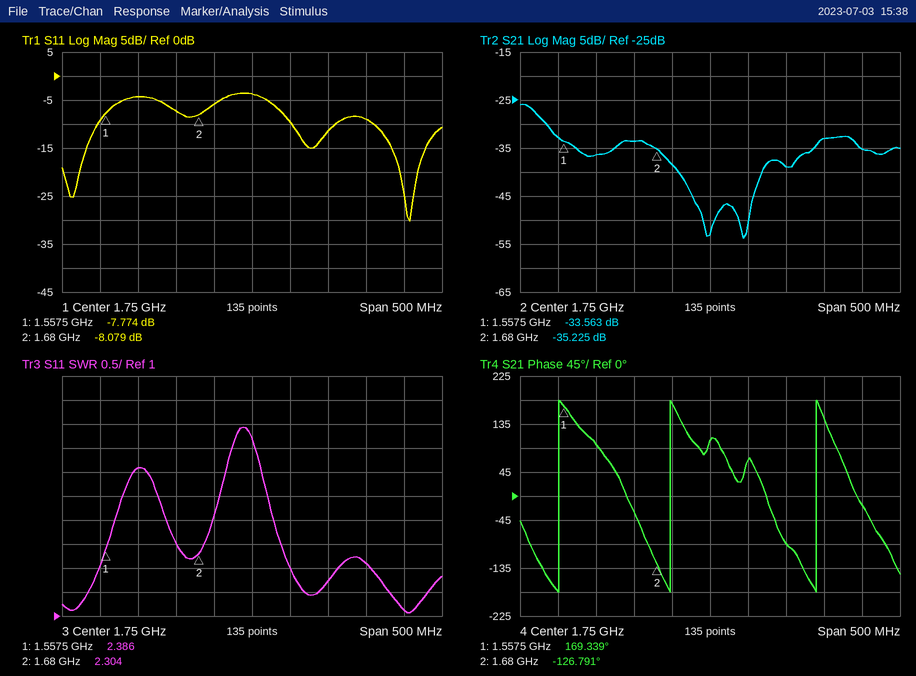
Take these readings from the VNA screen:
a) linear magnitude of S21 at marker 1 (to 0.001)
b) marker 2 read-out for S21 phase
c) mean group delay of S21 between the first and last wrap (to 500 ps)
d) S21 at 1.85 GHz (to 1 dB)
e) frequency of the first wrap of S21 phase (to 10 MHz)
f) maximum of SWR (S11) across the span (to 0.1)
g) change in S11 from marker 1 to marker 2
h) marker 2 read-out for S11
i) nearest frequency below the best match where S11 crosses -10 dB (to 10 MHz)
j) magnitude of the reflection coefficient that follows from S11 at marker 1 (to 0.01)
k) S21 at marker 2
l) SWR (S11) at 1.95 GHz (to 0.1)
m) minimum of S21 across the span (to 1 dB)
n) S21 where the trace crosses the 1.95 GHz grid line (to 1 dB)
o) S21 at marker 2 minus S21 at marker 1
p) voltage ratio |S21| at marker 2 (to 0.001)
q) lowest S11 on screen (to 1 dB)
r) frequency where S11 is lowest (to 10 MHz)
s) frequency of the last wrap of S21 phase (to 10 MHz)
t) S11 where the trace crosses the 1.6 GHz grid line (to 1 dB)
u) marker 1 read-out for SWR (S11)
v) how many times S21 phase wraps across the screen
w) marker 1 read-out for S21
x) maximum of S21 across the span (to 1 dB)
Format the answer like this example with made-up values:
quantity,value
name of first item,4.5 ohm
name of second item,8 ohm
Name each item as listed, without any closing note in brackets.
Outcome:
quantity,value
linear magnitude of S21 at marker 1,0.021
marker 2 read-out for S21 phase,-126.791°
mean group delay of S21 between the first and last wrap,6.0 ns
S21 at 1.85 GHz,-39 dB
frequency of the first wrap of S21 phase,1.55 GHz
maximum of SWR (S11) across the span,4.9
change in S11 from marker 1 to marker 2,-0.305 dB
marker 2 read-out for S11,-8.079 dB
nearest frequency below the best match where S11 crosses -10 dB,1.91 GHz
magnitude of the reflection coefficient that follows from S11 at marker 1,0.41
S21 at marker 2,-35.225 dB
SWR (S11) at 1.95 GHz,1.1
minimum of S21 across the span,-54 dB
S21 where the trace crosses the 1.95 GHz grid line,-35 dB
S21 at marker 2 minus S21 at marker 1,-1.662 dB
voltage ratio |S21| at marker 2,0.017
lowest S11 on screen,-30 dB
frequency where S11 is lowest,1.96 GHz
frequency of the last wrap of S21 phase,1.89 GHz
S11 where the trace crosses the 1.6 GHz grid line,-4 dB
marker 1 read-out for SWR,2.386
how many times S21 phase wraps across the screen,3
marker 1 read-out for S21,-33.563 dB
maximum of S21 across the span,-26 dB
